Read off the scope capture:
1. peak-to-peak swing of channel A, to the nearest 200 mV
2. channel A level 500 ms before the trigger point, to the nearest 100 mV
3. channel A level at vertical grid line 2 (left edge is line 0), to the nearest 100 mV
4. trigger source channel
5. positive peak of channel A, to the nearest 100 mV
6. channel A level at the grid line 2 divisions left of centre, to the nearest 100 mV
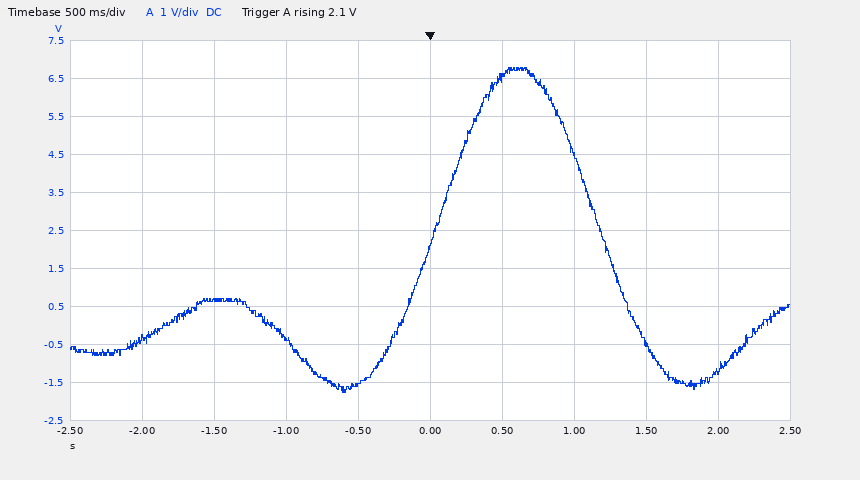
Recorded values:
8.6 V
-1.5 V
700 mV
channel A
6.8 V
-300 mV
